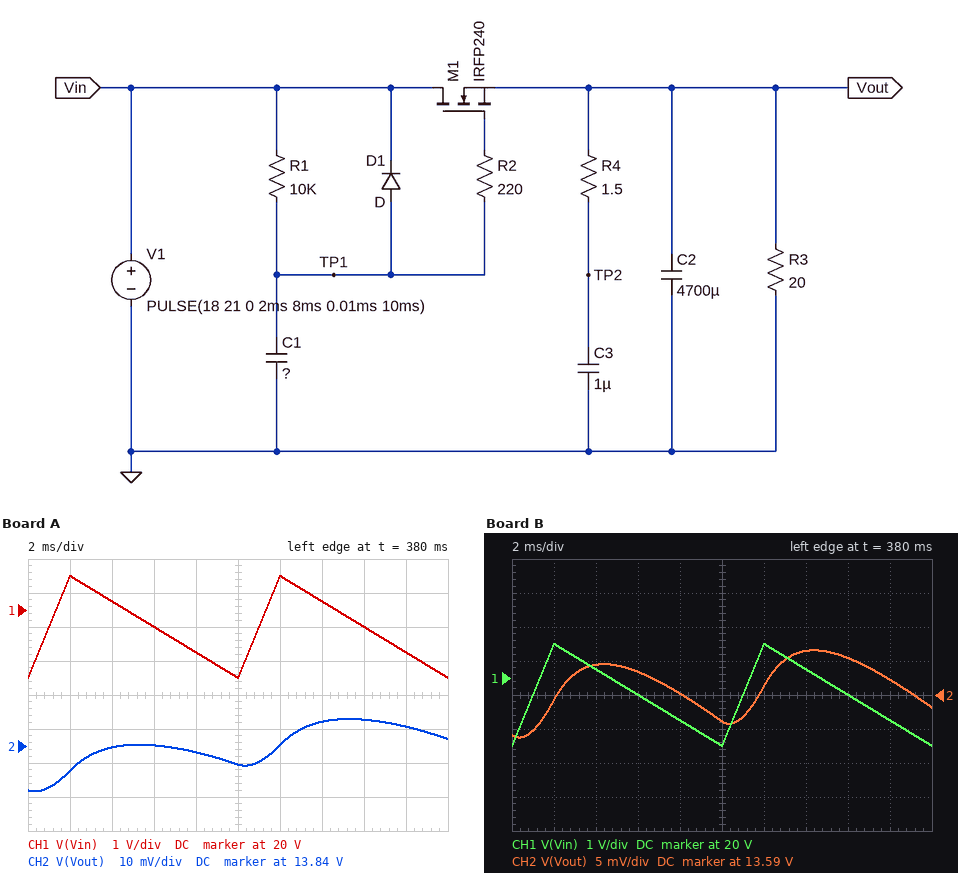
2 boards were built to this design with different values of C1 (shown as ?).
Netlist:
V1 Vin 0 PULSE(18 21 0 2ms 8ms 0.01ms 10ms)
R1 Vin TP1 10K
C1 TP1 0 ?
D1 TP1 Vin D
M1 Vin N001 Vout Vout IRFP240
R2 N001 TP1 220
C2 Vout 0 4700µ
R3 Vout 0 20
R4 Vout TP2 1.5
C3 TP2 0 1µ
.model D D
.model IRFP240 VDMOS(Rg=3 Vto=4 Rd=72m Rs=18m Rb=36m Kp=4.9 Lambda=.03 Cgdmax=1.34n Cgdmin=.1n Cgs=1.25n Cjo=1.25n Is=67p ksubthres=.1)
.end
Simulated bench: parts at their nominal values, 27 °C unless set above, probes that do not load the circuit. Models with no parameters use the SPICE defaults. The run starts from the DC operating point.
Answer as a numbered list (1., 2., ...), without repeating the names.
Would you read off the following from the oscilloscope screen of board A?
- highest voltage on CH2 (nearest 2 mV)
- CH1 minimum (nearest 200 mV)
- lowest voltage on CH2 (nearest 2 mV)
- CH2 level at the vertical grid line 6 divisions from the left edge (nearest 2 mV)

1. 13.848 V
2. 18.0 V
3. 13.826 V
4. 13.840 V
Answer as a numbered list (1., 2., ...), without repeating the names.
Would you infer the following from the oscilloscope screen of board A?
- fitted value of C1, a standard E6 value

1. 150 µF
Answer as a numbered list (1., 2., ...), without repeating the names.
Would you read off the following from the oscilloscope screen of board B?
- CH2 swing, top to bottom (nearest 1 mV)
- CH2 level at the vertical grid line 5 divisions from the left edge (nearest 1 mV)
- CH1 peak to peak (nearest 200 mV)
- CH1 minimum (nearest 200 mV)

1. 13 mV
2. 13.581 V
3. 3.0 V
4. 18.0 V
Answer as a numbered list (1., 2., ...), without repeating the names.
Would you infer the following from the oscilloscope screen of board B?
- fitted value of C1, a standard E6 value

1. 680 µF
